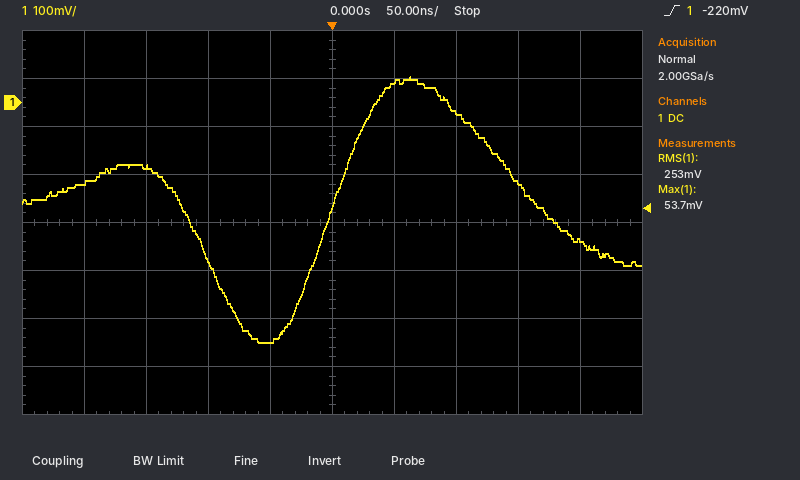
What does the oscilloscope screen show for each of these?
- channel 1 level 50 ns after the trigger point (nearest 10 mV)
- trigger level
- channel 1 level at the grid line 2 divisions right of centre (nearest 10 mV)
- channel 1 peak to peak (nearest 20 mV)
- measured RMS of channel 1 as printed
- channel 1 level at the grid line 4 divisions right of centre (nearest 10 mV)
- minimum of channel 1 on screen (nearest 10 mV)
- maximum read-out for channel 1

40 mV
-220 mV
-20 mV
560 mV
253 mV
-290 mV
-500 mV
53.7 mV
